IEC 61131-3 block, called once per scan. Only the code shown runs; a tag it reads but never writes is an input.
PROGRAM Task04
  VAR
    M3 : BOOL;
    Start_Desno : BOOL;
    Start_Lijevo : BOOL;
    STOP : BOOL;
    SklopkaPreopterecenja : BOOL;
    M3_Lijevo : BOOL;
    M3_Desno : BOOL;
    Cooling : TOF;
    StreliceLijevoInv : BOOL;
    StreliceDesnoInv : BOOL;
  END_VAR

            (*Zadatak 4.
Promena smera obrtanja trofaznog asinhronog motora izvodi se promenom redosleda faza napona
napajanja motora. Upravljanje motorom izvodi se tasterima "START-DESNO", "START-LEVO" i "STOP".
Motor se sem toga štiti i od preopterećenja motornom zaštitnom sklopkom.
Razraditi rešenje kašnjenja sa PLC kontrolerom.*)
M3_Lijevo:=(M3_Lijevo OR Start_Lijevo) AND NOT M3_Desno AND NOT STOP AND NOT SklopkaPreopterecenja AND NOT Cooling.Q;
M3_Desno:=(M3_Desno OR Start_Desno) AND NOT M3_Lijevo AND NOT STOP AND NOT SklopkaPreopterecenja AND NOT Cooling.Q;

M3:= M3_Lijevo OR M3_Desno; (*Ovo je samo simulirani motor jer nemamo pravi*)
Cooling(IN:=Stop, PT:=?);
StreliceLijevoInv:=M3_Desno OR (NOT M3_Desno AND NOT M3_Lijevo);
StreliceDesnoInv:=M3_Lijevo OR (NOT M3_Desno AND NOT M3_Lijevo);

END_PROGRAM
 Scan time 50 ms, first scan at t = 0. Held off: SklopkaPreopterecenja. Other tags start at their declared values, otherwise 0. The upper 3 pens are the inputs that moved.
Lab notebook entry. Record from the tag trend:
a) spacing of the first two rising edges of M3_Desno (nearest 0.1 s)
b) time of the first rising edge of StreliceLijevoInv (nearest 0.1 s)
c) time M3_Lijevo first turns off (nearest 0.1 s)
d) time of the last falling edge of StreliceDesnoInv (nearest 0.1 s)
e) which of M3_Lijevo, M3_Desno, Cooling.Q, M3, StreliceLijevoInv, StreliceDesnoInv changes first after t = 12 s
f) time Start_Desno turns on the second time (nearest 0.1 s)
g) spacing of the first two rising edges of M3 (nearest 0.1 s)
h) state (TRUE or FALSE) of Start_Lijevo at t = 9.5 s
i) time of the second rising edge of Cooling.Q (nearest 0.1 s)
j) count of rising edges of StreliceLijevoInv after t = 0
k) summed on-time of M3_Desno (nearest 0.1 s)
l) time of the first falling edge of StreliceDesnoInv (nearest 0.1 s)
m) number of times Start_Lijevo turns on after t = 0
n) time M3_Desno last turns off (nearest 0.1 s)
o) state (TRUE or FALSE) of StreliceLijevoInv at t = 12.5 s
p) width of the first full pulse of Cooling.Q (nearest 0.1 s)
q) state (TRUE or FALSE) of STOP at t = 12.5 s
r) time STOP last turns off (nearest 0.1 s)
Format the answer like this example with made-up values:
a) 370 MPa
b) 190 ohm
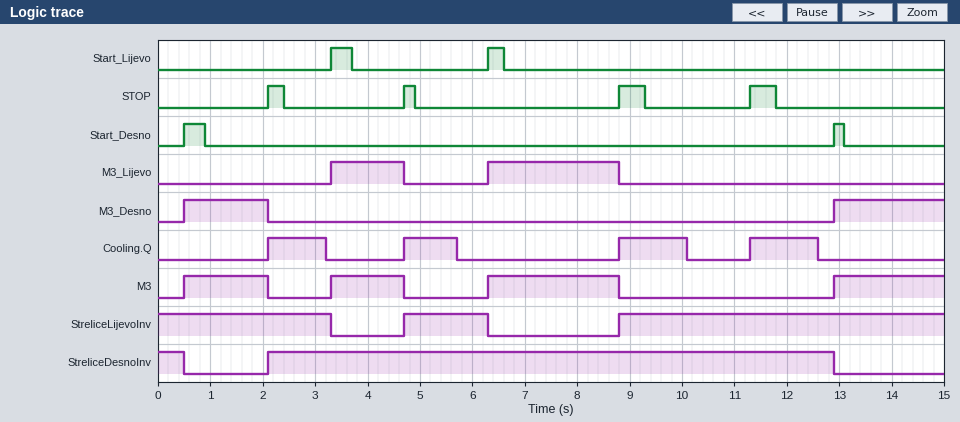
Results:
a) 12.4 s
b) 4.7 s
c) 4.7 s
d) 12.9 s
e) Cooling.Q
f) 12.9 s
g) 2.8 s
h) FALSE
i) 4.7 s
j) 2
k) 3.7 s
l) 0.5 s
m) 2
n) 2.1 s
o) TRUE
p) 1.1 s
q) FALSE
r) 11.8 s
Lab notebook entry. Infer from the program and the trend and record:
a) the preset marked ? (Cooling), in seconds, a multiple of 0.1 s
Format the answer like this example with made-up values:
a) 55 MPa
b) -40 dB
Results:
a) 0.8 s
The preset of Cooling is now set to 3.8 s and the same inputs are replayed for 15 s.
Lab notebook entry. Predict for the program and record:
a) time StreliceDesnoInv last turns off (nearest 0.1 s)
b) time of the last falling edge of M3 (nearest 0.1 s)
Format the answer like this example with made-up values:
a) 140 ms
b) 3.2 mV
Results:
a) 0.5 s
b) 2.1 s
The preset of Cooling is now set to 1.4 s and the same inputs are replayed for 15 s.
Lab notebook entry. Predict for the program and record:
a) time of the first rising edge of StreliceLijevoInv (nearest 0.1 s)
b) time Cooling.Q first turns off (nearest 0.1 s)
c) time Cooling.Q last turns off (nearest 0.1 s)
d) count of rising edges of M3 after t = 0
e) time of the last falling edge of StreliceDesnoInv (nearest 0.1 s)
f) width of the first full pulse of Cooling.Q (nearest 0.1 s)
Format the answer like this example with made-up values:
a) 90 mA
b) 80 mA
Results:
a) 8.8 s
b) 3.8 s
c) 13.2 s
d) 2
e) 0.5 s
f) 1.7 s
